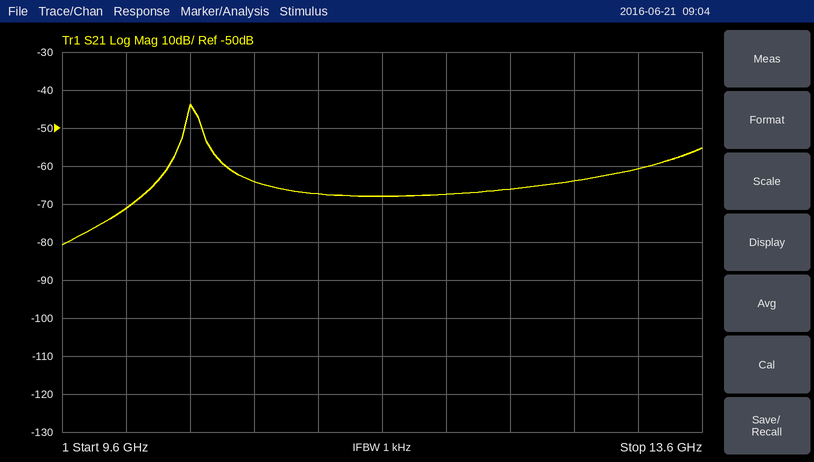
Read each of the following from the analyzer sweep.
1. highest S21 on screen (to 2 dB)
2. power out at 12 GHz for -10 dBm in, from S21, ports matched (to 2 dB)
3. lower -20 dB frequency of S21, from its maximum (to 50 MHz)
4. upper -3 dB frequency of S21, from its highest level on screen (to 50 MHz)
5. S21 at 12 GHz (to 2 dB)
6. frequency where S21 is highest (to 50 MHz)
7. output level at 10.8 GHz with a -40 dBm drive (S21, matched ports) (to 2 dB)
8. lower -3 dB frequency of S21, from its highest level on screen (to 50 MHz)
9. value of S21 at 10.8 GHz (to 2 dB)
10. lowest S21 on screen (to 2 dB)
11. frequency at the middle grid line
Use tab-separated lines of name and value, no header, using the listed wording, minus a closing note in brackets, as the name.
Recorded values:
highest S21 on screen	-44 dB
power out at 12 GHz for -10 dBm in, from S21, ports matched	-78 dBm
lower -20 dB frequency of S21, from its maximum	10.20 GHz
upper -3 dB frequency of S21, from its highest level on screen	10.45 GHz
S21 at 12 GHz	-68 dB
frequency where S21 is highest	10.40 GHz
output level at 10.8 GHz with a -40 dBm drive (S21, matched ports)	-104 dBm
lower -3 dB frequency of S21, from its highest level on screen	10.40 GHz
value of S21 at 10.8 GHz	-64 dB
lowest S21 on screen	-80 dB
frequency at the middle grid line	11.6 GHz
